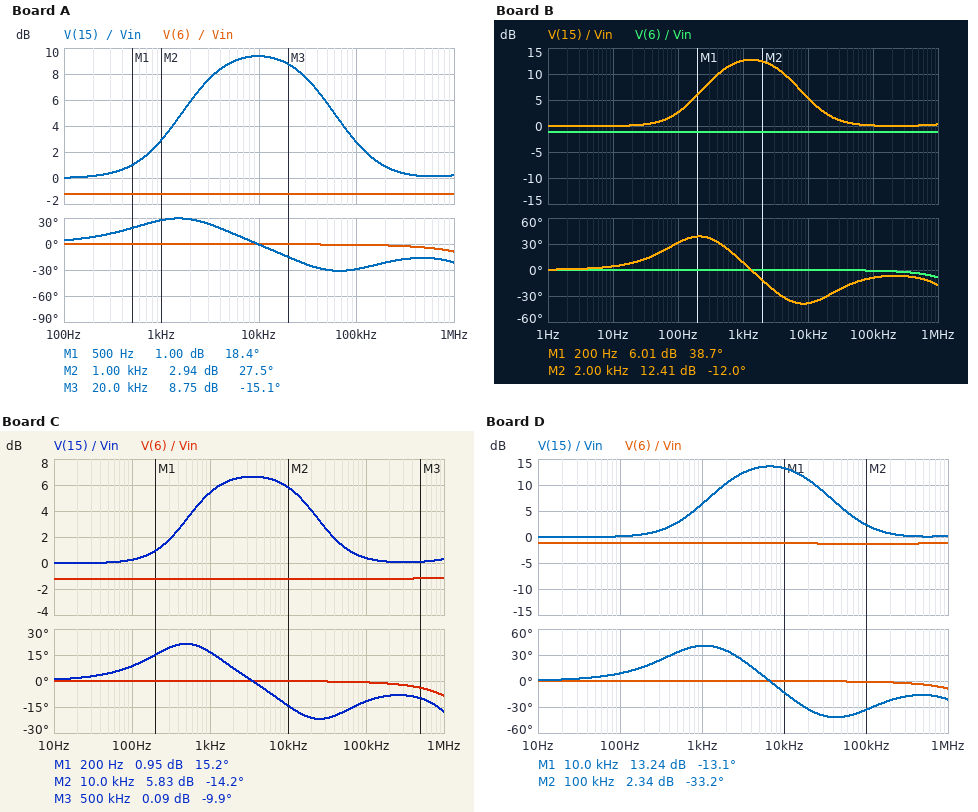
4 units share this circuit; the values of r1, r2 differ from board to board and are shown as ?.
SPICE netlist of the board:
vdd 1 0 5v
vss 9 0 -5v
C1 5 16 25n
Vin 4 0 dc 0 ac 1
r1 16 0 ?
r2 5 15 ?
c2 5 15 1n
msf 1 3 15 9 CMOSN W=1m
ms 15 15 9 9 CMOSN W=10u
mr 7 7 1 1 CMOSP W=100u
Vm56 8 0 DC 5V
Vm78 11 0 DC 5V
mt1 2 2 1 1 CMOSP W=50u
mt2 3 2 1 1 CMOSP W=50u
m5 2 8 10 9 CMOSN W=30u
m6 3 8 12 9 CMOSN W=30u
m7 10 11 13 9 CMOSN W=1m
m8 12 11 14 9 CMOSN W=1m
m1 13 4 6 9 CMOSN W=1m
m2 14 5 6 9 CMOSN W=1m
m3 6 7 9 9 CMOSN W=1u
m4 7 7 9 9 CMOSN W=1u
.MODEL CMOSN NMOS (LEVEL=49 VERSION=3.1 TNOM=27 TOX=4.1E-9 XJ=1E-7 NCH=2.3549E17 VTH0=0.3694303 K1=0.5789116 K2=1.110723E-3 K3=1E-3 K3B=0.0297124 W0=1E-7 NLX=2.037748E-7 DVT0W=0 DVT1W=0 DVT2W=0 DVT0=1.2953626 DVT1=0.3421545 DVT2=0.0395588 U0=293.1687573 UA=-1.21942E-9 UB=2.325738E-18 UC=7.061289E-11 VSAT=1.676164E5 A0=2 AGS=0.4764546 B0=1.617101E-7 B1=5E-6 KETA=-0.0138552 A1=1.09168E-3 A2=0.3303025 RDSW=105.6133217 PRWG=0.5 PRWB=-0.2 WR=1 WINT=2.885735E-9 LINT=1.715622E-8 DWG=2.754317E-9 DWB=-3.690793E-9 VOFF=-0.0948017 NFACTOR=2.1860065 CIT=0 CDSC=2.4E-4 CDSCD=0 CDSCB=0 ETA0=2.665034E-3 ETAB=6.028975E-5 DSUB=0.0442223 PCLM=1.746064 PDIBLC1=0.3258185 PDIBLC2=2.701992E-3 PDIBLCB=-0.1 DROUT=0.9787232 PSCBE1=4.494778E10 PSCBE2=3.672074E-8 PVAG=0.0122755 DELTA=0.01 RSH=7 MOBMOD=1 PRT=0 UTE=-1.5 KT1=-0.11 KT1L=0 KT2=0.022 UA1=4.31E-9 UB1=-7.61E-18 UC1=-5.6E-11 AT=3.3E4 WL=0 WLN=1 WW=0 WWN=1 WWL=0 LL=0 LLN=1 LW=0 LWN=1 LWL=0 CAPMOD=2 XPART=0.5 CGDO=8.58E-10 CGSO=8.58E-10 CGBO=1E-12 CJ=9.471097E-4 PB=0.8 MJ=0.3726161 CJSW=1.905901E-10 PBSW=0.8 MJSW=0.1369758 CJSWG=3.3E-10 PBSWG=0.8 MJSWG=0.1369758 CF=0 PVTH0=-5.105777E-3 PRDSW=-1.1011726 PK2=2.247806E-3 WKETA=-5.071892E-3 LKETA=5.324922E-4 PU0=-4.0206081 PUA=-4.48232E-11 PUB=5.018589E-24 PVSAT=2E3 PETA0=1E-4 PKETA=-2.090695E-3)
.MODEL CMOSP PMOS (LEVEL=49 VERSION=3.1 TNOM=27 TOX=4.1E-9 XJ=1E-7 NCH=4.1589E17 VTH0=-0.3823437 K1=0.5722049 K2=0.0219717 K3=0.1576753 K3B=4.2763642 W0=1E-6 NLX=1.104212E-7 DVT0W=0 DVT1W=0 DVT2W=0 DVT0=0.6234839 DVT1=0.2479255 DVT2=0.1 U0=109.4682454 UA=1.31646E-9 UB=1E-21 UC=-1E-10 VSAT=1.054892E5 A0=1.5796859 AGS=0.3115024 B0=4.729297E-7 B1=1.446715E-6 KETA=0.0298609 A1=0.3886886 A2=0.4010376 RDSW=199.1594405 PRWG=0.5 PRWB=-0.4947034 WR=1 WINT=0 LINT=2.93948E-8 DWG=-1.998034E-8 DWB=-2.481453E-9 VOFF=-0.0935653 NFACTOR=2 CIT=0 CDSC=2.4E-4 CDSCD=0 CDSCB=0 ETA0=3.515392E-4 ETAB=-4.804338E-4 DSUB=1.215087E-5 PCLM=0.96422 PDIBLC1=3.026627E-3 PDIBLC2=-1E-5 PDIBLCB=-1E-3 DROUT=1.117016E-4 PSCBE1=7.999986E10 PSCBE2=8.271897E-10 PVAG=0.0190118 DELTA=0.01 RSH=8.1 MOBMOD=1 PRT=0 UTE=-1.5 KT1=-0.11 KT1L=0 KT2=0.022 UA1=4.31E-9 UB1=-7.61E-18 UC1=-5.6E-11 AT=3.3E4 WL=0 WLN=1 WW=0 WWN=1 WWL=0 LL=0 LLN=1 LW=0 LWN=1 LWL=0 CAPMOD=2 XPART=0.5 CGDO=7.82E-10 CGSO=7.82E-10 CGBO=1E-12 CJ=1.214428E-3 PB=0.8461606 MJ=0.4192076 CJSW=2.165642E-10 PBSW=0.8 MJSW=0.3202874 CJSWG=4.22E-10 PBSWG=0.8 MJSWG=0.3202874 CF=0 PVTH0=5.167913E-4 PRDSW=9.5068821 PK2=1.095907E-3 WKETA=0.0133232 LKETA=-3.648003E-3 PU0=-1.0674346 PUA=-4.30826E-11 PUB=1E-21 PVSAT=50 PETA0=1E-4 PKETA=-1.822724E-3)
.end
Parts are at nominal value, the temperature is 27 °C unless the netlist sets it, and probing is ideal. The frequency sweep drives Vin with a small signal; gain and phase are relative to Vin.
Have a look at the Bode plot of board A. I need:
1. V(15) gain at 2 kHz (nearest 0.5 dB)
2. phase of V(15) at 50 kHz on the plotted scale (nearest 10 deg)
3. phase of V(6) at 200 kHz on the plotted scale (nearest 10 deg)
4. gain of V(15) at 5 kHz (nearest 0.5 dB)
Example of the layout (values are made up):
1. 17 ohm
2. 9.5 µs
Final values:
1. 6.0 dB
2. -30 deg
3. 0 deg
4. 9.0 dB
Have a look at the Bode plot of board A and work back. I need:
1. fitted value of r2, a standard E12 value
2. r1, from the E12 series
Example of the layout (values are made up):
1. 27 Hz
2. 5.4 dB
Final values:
1. 4.7 kΩ
2. 2.2 kΩ
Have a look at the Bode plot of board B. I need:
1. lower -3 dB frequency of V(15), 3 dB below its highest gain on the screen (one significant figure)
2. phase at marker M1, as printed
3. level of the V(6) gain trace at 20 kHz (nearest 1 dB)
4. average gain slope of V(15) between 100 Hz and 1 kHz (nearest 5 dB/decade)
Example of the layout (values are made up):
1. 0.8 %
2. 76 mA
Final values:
1. 400 Hz
2. 38.7 deg
3. -1 dB
4. 10 dB/decade
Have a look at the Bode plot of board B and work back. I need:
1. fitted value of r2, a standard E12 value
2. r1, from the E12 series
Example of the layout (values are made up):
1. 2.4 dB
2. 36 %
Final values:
1. 47 kΩ
2. 12 kΩ
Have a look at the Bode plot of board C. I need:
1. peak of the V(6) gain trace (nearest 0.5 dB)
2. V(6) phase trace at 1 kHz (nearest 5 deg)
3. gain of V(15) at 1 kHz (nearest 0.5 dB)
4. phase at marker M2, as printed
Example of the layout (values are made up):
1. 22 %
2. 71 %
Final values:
1. -1.0 dB
2. 0 deg
3. 5.5 dB
4. -14.2 deg
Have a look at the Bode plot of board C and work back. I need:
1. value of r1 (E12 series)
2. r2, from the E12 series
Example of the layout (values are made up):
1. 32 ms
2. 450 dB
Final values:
1. 8.2 kΩ
2. 10 kΩ
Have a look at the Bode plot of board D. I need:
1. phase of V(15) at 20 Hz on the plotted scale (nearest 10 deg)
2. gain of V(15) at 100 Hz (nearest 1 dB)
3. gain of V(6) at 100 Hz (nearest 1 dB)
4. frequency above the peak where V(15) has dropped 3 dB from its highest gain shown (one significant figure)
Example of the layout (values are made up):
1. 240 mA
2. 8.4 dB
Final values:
1. 0 deg
2. 0 dB
3. -1 dB
4. 20 kHz
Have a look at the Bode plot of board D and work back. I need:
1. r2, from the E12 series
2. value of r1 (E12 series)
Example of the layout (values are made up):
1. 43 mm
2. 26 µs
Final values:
1. 10 kΩ
2. 2.2 kΩ
